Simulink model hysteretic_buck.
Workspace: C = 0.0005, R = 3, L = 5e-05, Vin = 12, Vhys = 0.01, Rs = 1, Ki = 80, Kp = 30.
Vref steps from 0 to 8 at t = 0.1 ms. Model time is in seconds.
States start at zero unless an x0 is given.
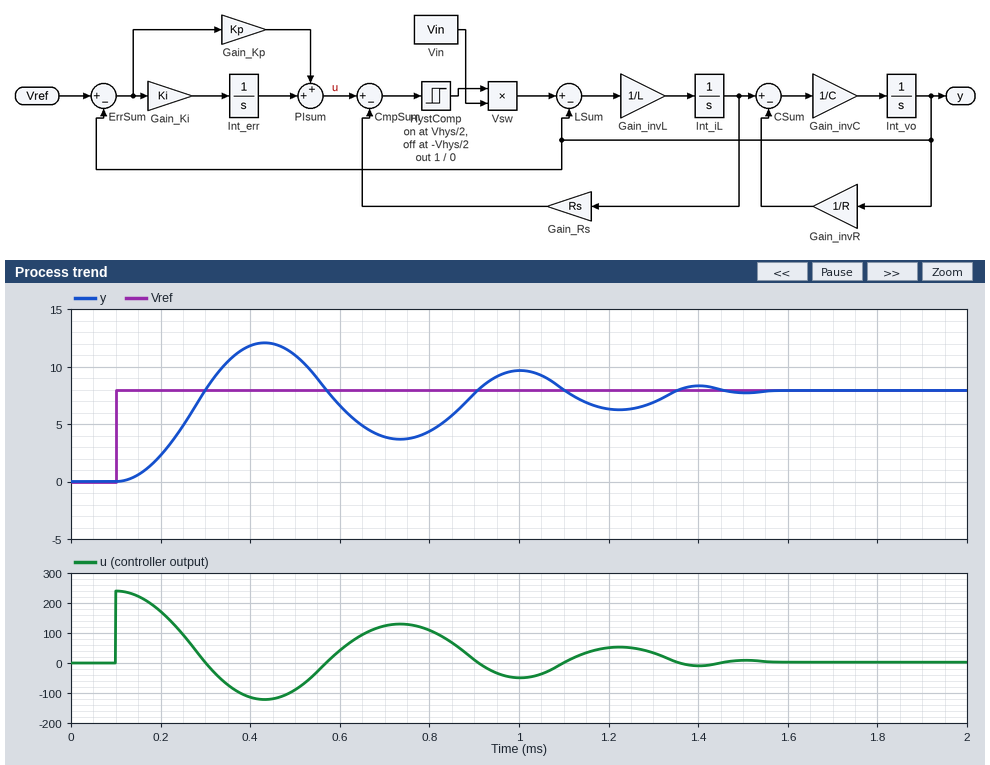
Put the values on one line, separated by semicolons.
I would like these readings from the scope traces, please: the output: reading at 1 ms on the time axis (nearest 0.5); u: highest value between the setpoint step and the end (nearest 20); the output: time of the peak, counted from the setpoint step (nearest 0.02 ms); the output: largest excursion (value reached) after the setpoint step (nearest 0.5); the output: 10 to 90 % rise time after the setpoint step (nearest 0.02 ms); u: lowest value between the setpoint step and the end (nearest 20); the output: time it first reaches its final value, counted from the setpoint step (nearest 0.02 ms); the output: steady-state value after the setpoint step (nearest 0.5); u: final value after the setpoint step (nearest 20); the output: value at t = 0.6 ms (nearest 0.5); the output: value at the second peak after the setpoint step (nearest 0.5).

9.5; 240; 0.34 ms; 12.0; 0.12 ms; -120; 0.20 ms; 8.0; 0; 6.5; 9.5
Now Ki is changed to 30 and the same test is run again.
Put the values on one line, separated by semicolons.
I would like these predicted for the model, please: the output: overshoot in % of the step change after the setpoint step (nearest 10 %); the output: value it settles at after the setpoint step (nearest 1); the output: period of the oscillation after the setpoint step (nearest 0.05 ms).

50 %; 8; 0.55 ms
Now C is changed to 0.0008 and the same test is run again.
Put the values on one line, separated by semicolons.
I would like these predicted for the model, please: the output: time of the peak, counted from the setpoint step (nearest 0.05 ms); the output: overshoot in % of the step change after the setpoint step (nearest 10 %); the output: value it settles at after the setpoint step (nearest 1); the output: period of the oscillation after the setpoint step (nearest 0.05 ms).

0.40 ms; 50 %; 8; 0.70 ms
